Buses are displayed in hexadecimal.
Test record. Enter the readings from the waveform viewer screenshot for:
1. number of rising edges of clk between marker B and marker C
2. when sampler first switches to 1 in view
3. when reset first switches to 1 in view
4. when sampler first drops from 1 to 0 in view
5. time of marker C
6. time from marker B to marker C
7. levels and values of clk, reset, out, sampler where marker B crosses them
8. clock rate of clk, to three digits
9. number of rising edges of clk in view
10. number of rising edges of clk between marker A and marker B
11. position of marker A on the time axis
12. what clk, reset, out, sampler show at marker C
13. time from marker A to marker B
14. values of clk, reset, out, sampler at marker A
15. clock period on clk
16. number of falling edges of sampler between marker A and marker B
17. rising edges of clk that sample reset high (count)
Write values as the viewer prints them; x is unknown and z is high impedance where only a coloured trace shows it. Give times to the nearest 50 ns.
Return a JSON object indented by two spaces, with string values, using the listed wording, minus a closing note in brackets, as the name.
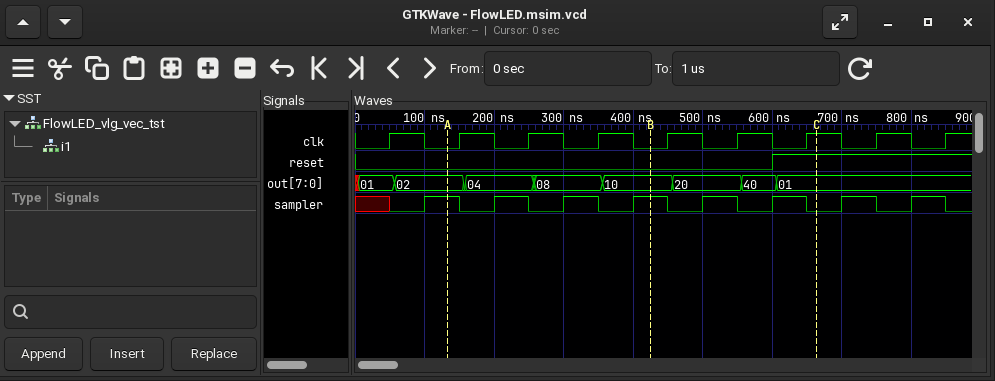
{
  "number of rising edges of clk between marker B and marker C": "3",
  "when sampler first switches to 1 in view": "100 ns",
  "when reset first switches to 1 in view": "600 ns",
  "when sampler first drops from 1 to 0 in view": "150 ns",
  "time of marker C": "650 ns",
  "time from marker B to marker C": "250 ns",
  "levels and values of clk, reset, out, sampler where marker B crosses them": "clk=0, reset=0, out=10, sampler=1",
  "clock rate of clk, to three digits": "10.0 MHz",
  "number of rising edges of clk in view": "9",
  "number of rising edges of clk between marker A and marker B": "3",
  "position of marker A on the time axis": "150 ns",
  "what clk, reset, out, sampler show at marker C": "clk=1, reset=1, out=01, sampler=0",
  "time from marker A to marker B": "300 ns",
  "values of clk, reset, out, sampler at marker A": "clk=0, reset=0, out=02, sampler=1",
  "clock period on clk": "100 ns",
  "number of falling edges of sampler between marker A and marker B": "3",
  "rising edges of clk that sample reset high": "3"
}
